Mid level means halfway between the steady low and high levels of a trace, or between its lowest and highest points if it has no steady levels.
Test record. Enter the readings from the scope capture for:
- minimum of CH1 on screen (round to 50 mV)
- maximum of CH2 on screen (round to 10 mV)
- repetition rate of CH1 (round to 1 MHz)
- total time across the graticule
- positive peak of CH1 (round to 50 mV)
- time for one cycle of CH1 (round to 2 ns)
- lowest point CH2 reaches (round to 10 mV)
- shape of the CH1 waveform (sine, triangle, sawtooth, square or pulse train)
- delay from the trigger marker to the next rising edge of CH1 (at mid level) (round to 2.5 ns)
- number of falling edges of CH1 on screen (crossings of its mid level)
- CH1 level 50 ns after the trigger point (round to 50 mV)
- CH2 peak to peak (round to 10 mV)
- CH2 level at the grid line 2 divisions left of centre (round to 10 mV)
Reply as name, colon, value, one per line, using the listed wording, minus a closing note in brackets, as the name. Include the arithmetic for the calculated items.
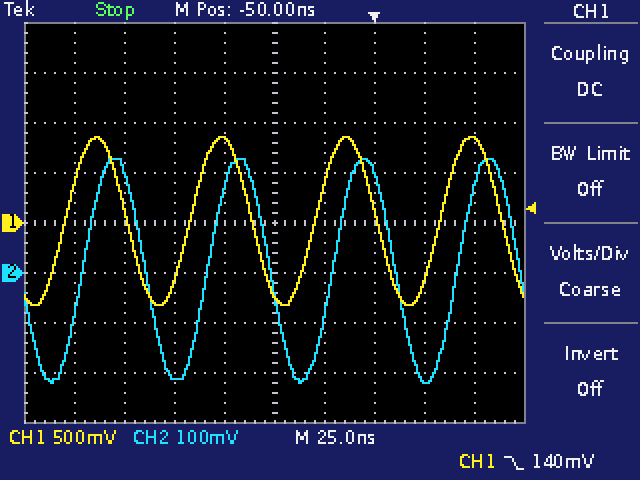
minimum of CH1 on screen: -800 mV
maximum of CH2 on screen: 230 mV
repetition rate of CH1: 1 / 62 ns ≈ 16 MHz
total time across the graticule: 250 ns
positive peak of CH1: 850 mV
time for one cycle of CH1: 62 ns
lowest point CH2 reaches: -220 mV
shape of the CH1 waveform: sine
delay from the trigger marker to the next rising edge of CH1 (at mid level): 32.5 ns
number of falling edges of CH1 on screen: 4
CH1 level 50 ns after the trigger point: 850 mV
CH2 peak to peak: 230 mV − (-220 mV) = 450 mV
CH2 level at the grid line 2 divisions left of centre: -210 mV
